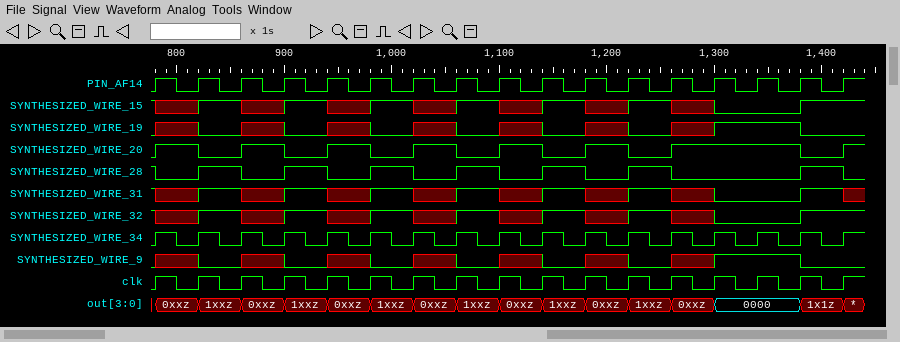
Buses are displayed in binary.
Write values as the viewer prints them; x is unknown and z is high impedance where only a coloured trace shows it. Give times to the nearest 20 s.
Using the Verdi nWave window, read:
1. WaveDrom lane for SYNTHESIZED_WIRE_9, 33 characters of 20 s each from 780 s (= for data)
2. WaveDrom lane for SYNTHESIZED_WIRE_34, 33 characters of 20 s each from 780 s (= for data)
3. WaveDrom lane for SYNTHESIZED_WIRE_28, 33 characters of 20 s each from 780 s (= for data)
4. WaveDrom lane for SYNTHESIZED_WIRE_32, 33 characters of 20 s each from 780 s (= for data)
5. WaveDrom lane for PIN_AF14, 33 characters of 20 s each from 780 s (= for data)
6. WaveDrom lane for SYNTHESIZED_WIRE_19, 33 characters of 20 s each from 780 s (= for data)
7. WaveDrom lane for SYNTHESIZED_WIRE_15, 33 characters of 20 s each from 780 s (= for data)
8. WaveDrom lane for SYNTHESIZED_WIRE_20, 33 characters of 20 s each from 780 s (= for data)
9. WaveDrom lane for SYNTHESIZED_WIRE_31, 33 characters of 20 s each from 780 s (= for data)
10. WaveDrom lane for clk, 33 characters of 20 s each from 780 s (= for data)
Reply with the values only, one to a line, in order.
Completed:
{name: 'SYNTHESIZED_WIRE_9', wave: 'x.0.x.0.x.0.x.0.x.0.x.0.x.1...0..'}
{name: 'SYNTHESIZED_WIRE_34', wave: '101010101010101010101010101010101'}
{name: 'SYNTHESIZED_WIRE_28', wave: '0.1.0.1.0.1.0.1.0.1.0.1.0.....1.0'}
{name: 'SYNTHESIZED_WIRE_32', wave: 'x.1.x.1.x.1.x.1.x.1.x.1.x.0...1..'}
{name: 'PIN_AF14', wave: '101010101010101010101010101010101'}
{name: 'SYNTHESIZED_WIRE_19', wave: 'x.0.x.0.x.0.x.0.x.0.x.0.x.1...0..'}
{name: 'SYNTHESIZED_WIRE_15', wave: 'x.1.x.1.x.1.x.1.x.1.x.1.x.0...1..'}
{name: 'SYNTHESIZED_WIRE_20', wave: '1.0.1.0.1.0.1.0.1.0.1.0.1.....0.1'}
{name: 'SYNTHESIZED_WIRE_31', wave: 'x.1.x.1.x.1.x.1.x.1.x.1.x.0...1.x'}
{name: 'clk', wave: '101010101010101010101010101010101'}
